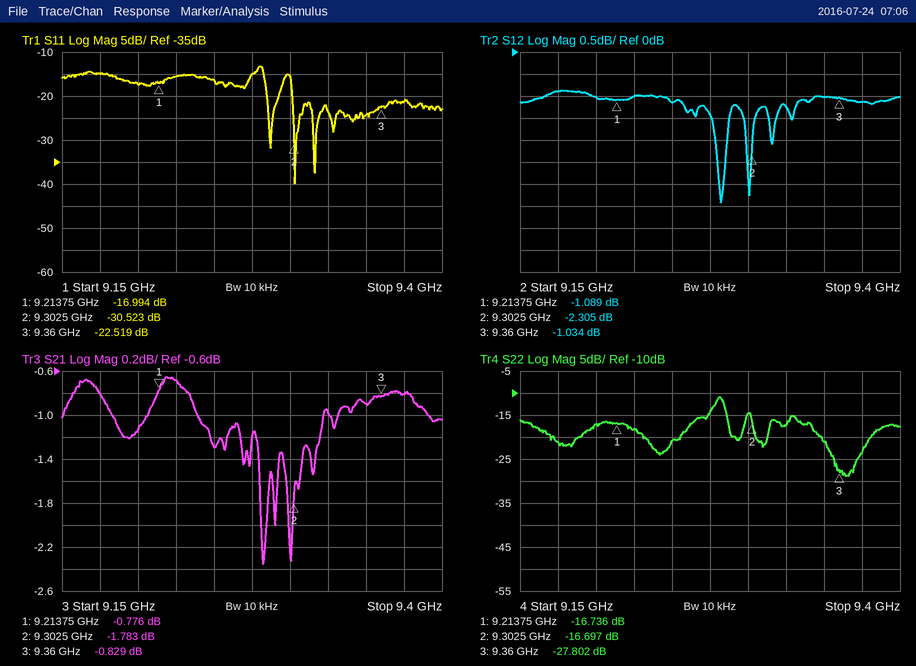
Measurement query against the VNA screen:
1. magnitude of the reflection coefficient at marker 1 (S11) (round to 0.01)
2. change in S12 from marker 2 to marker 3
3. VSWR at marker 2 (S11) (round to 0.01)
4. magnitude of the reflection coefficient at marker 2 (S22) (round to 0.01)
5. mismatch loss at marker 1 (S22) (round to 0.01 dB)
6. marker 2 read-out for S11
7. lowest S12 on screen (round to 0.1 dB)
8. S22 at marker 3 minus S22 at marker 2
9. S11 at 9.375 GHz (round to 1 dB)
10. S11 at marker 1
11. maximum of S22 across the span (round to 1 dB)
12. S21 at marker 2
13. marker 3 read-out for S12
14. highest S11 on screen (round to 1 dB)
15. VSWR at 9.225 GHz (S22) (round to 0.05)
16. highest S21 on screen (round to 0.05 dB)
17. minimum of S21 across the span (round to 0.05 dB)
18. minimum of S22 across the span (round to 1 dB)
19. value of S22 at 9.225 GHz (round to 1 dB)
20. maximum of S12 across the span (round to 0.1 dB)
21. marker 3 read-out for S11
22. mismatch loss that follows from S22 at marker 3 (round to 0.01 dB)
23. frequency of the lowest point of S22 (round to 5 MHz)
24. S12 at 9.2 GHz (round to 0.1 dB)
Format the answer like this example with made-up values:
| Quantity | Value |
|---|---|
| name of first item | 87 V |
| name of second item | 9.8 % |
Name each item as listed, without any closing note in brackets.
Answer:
| Quantity | Value |
|---|---|
| magnitude of the reflection coefficient at marker 1 (S11) | 0.14 |
| change in S12 from marker 2 to marker 3 | 1.271 dB |
| VSWR at marker 2 (S11) | 1.06 |
| magnitude of the reflection coefficient at marker 2 (S22) | 0.15 |
| mismatch loss at marker 1 (S22) | 0.09 dB |
| marker 2 read-out for S11 | -30.523 dB |
| lowest S12 on screen | -3.4 dB |
| S22 at marker 3 minus S22 at marker 2 | -11.105 dB |
| S11 at 9.375 GHz | -21 dB |
| S11 at marker 1 | -16.994 dB |
| maximum of S22 across the span | -11 dB |
| S21 at marker 2 | -1.783 dB |
| marker 3 read-out for S12 | -1.034 dB |
| highest S11 on screen | -13 dB |
| VSWR at 9.225 GHz (S22) | 1.30 |
| highest S21 on screen | -0.65 dB |
| minimum of S21 across the span | -2.35 dB |
| minimum of S22 across the span | -29 dB |
| value of S22 at 9.225 GHz | -18 dB |
| maximum of S12 across the span | -0.9 dB |
| marker 3 read-out for S11 | -22.519 dB |
| mismatch loss that follows from S22 at marker 3 | 0.01 dB |
| frequency of the lowest point of S22 | 9.365 GHz |
| S12 at 9.2 GHz | -1.0 dB |
